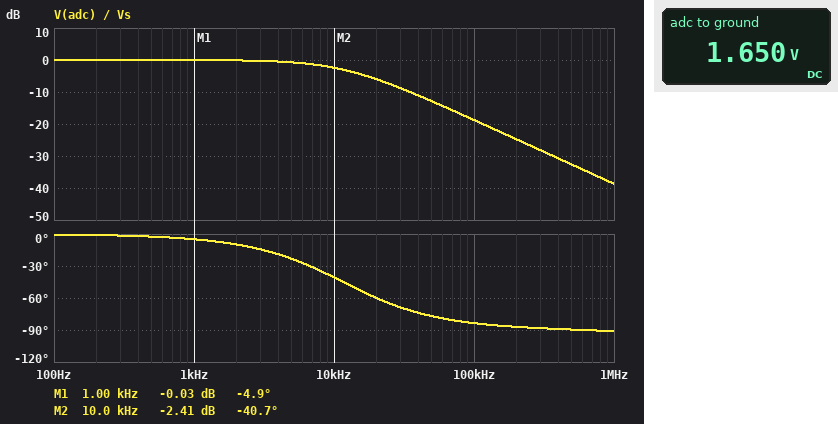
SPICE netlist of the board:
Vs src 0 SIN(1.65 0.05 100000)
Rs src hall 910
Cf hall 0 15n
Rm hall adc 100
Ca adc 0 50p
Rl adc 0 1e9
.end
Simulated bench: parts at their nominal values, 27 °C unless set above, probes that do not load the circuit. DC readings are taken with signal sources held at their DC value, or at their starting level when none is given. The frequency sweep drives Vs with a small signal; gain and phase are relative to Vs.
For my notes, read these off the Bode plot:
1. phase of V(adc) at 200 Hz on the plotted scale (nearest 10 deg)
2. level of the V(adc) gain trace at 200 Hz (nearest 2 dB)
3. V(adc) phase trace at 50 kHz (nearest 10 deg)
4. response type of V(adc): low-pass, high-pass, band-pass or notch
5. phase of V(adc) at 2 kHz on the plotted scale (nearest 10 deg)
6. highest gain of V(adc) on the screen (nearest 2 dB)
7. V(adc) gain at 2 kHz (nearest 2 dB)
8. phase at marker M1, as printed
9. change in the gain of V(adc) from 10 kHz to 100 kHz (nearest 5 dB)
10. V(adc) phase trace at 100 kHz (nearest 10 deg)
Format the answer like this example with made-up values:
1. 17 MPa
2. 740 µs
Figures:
1. 0 deg
2. 0 dB
3. -80 deg
4. low-pass
5. -10 deg
6. 0 dB
7. 0 dB
8. -4.9 deg
9. -15 dB
10. -80 deg
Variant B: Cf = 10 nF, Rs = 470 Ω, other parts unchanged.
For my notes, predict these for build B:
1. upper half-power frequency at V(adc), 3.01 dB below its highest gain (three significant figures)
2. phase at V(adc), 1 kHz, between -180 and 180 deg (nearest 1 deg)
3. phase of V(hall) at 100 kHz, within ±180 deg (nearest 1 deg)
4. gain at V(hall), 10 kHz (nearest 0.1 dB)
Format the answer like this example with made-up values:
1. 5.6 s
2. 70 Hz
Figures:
1. 33.7 kHz
2. -2 deg
3. -71 deg
4. -0.4 dB
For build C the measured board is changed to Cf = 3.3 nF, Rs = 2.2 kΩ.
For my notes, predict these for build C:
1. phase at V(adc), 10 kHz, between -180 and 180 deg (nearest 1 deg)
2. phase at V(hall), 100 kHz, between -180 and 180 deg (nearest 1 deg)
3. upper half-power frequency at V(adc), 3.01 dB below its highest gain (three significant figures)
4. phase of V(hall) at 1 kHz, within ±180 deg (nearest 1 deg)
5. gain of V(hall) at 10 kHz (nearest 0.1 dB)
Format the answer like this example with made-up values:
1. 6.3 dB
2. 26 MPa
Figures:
1. -25 deg
2. -78 deg
3. 21.6 kHz
4. -3 deg
5. -0.8 dB
